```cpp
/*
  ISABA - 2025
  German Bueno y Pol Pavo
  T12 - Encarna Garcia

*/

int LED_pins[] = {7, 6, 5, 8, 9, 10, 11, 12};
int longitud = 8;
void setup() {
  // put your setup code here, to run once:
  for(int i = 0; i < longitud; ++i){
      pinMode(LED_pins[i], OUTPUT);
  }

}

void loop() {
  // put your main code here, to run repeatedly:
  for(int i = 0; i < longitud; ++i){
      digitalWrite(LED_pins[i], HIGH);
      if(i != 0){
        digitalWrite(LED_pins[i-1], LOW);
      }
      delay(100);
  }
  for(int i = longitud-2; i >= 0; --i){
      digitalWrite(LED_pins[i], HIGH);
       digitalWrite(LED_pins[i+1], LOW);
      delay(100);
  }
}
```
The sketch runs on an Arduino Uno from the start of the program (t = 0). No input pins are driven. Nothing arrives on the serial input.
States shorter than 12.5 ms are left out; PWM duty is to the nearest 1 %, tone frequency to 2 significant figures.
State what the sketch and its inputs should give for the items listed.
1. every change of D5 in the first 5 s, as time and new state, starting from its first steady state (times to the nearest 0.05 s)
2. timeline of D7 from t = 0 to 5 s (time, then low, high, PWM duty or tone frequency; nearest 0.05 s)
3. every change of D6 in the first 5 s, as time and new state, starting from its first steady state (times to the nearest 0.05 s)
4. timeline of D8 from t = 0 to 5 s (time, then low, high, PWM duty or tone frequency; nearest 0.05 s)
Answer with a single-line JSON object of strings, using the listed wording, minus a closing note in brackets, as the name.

{"every change of D5 in the first 5 s, as time and new state, starting from its first steady state": "0 s low; 0.2 s high; 0.3 s low; 1.2 s high; 1.3 s low; 1.7 s high; 1.8 s low; 2.7 s high; 2.8 s low; 3.2 s high; 3.3 s low; 4.2 s high; 4.3 s low; 4.7 s high; 4.8 s low", "timeline of D7 from t = 0 to 5 s": "0 s high; 0.1 s low; 1.4 s high; 1.6 s low; 2.9 s high; 3.1 s low; 4.4 s high; 4.6 s low", "every change of D6 in the first 5 s, as time and new state, starting from its first steady state": "0 s low; 0.1 s high; 0.2 s low; 1.3 s high; 1.4 s low; 1.6 s high; 1.7 s low; 2.8 s high; 2.9 s low; 3.1 s high; 3.2 s low; 4.3 s high; 4.4 s low; 4.6 s high; 4.7 s low", "timeline of D8 from t = 0 to 5 s": "0 s low; 0.3 s high; 0.4 s low; 1.1 s high; 1.2 s low; 1.8 s high; 1.9 s low; 2.6 s high; 2.7 s low; 3.3 s high; 3.4 s low; 4.1 s high; 4.2 s low; 4.8 s high; 4.9 s low"}
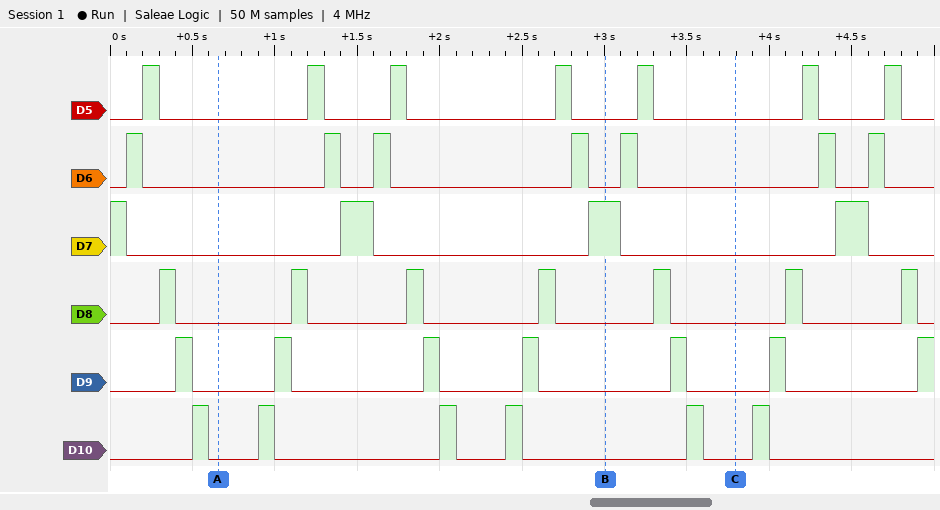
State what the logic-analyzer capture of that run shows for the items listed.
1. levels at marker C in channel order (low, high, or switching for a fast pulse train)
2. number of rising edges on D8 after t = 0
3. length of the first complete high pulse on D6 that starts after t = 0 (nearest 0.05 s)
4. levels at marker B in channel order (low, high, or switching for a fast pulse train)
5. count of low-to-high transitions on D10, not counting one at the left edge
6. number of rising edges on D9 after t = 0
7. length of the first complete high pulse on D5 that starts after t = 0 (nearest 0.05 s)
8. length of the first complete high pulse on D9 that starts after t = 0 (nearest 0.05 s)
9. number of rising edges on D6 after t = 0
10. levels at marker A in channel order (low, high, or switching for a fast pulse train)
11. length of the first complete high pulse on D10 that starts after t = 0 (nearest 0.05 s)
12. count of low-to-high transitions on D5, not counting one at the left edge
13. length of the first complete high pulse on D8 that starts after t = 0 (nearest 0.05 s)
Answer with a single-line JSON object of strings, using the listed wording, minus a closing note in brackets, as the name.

{"levels at marker C in channel order": "D5 low, D6 low, D7 low, D8 low, D9 low, D10 low", "number of rising edges on D8 after t = 0": "7", "length of the first complete high pulse on D6 that starts after t = 0": "0.10 s", "levels at marker B in channel order": "D5 low, D6 low, D7 high, D8 low, D9 low, D10 low", "count of low-to-high transitions on D10, not counting one at the left edge": "6", "number of rising edges on D9 after t = 0": "7", "length of the first complete high pulse on D5 that starts after t = 0": "0.10 s", "length of the first complete high pulse on D9 that starts after t = 0": "0.10 s", "number of rising edges on D6 after t = 0": "7", "levels at marker A in channel order": "D5 low, D6 low, D7 low, D8 low, D9 low, D10 low", "length of the first complete high pulse on D10 that starts after t = 0": "0.10 s", "count of low-to-high transitions on D5, not counting one at the left edge": "7", "length of the first complete high pulse on D8 that starts after t = 0": "0.10 s"}
